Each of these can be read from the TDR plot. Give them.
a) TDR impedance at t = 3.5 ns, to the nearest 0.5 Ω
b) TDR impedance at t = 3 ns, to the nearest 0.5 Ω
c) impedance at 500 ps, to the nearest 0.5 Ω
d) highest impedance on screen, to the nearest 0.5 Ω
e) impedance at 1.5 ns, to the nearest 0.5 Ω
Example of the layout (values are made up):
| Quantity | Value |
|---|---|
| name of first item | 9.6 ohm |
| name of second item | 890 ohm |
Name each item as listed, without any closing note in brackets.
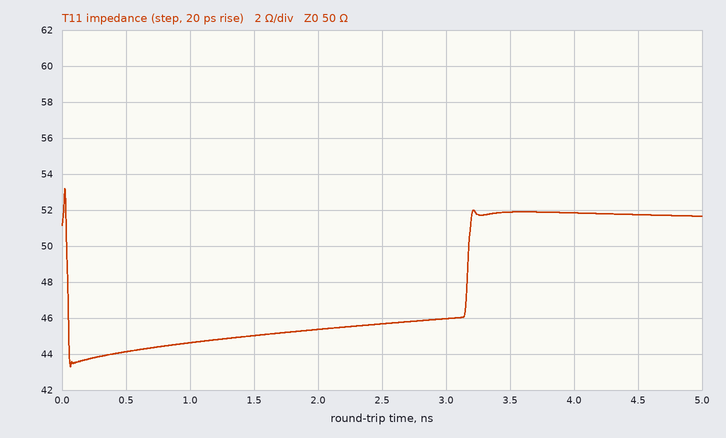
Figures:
| Quantity | Value |
|---|---|
| TDR impedance at t = 3.5 ns, to the nearest 0.5 Ω | 52.0 Ω |
| TDR impedance at t = 3 ns, to the nearest 0.5 Ω | 46.0 Ω |
| impedance at 500 ps, to the nearest 0.5 Ω | 44.0 Ω |
| highest impedance on screen, to the nearest 0.5 Ω | 53.0 Ω |
| impedance at 1.5 ns, to the nearest 0.5 Ω | 45.0 Ω |
